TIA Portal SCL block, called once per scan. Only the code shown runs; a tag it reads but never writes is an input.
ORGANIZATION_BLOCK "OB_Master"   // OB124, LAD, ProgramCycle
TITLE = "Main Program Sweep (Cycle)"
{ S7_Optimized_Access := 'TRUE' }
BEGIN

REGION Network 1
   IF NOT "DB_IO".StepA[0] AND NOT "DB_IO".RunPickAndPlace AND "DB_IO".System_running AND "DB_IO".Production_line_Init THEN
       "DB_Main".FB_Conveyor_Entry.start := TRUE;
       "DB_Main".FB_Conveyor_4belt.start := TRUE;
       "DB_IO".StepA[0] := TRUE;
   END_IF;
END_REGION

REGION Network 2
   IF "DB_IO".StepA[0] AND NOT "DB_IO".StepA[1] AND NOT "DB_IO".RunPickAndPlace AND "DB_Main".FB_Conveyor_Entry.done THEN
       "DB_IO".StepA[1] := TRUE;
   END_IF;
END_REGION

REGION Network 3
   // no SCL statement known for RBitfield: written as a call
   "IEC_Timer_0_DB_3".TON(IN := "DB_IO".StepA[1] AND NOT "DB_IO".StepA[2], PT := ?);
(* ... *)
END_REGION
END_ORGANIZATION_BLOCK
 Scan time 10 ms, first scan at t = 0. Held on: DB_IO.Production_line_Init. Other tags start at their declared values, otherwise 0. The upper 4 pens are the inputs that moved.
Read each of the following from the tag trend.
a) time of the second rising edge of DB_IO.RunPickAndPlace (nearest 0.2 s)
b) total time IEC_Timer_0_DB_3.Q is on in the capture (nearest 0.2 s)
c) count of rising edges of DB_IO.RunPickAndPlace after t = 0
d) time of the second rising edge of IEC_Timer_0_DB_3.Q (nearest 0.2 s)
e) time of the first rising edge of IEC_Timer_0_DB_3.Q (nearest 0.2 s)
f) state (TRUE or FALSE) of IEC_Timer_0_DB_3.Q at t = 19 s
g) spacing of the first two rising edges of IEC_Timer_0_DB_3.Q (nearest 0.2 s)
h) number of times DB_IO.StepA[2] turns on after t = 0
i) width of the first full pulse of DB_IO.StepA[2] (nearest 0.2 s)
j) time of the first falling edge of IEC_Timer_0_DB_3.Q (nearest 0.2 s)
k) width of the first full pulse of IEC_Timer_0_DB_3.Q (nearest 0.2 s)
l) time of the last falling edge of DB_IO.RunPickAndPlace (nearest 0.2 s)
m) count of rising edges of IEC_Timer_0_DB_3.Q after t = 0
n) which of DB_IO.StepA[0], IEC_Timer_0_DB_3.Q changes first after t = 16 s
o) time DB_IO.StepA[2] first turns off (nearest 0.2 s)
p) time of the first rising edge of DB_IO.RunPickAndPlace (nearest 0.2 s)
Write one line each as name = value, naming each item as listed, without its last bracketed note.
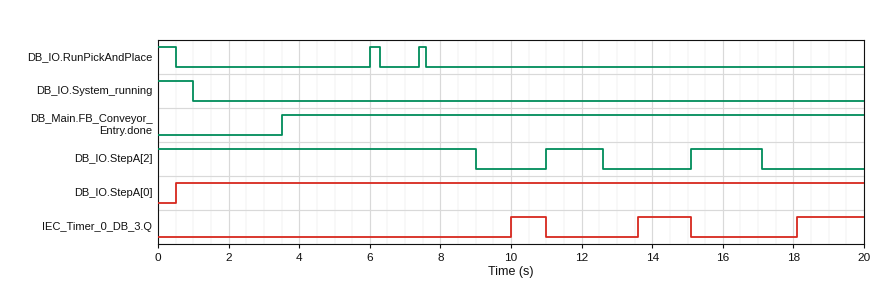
time of the second rising edge of DB_IO.RunPickAndPlace = 7.4 s
total time IEC_Timer_0_DB_3.Q is on in the capture = 4.4 s
count of rising edges of DB_IO.RunPickAndPlace after t = 0 = 2
time of the second rising edge of IEC_Timer_0_DB_3.Q = 13.6 s
time of the first rising edge of IEC_Timer_0_DB_3.Q = 10.0 s
state (TRUE or FALSE) of IEC_Timer_0_DB_3.Q at t = 19 s = TRUE
spacing of the first two rising edges of IEC_Timer_0_DB_3.Q = 3.6 s
number of times DB_IO.StepA[2] turns on after t = 0 = 2
width of the first full pulse of DB_IO.StepA[2] = 1.6 s
time of the first falling edge of IEC_Timer_0_DB_3.Q = 11.0 s
width of the first full pulse of IEC_Timer_0_DB_3.Q = 1.0 s
time of the last falling edge of DB_IO.RunPickAndPlace = 7.6 s
count of rising edges of IEC_Timer_0_DB_3.Q after t = 0 = 3
which of DB_IO.StepA[0], IEC_Timer_0_DB_3.Q changes first after t = 16 s = IEC_Timer_0_DB_3.Q
time DB_IO.StepA[2] first turns off = 9.0 s
time of the first rising edge of DB_IO.RunPickAndPlace = 6.0 s
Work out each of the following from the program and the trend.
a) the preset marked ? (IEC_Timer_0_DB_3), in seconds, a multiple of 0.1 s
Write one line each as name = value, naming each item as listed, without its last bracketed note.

the preset marked ? (IEC_Timer_0_DB_3), in seconds, a multiple of 0.1 s = 1.0 s
